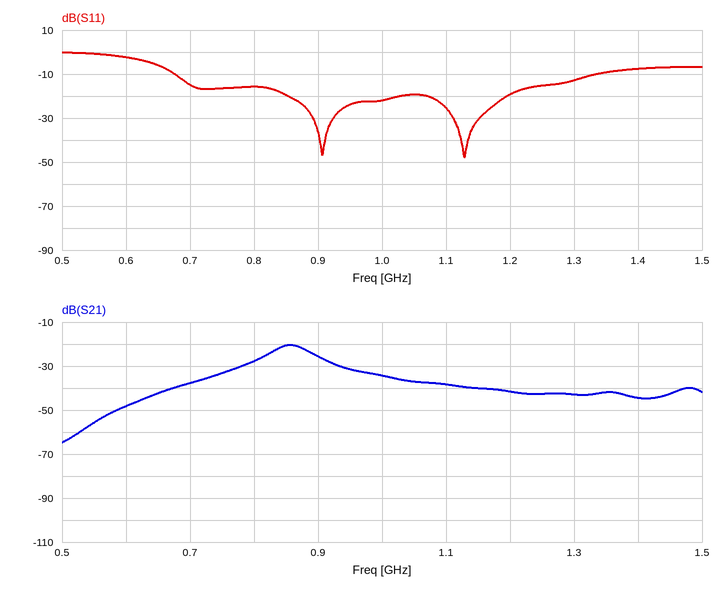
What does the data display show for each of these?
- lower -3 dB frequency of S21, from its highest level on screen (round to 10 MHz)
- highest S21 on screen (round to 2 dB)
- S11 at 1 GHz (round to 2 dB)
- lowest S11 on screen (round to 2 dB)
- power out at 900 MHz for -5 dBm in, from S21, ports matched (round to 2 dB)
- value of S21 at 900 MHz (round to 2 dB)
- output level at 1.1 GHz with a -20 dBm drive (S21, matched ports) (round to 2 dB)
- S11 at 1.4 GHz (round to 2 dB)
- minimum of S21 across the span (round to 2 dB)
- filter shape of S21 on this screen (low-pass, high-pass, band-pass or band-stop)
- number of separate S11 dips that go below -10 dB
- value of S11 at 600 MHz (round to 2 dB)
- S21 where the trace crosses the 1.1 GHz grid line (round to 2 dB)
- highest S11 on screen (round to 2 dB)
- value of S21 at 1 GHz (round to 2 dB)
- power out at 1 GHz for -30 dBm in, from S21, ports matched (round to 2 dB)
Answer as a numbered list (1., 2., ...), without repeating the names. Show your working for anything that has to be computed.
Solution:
1. 830 MHz
2. -20 dB
3. -22 dB
4. -48 dB
5. -5 dBm + (-26 dB) = -30 dBm
6. -26 dB
7. -20 dBm + (-38 dB) = -58 dBm
8. -8 dB
9. -64 dB
10. band-pass
11. 2
12. -2 dB
13. -38 dB
14. 0 dB
15. -34 dB
16. -30 dBm + (-34 dB) = -64 dBm
